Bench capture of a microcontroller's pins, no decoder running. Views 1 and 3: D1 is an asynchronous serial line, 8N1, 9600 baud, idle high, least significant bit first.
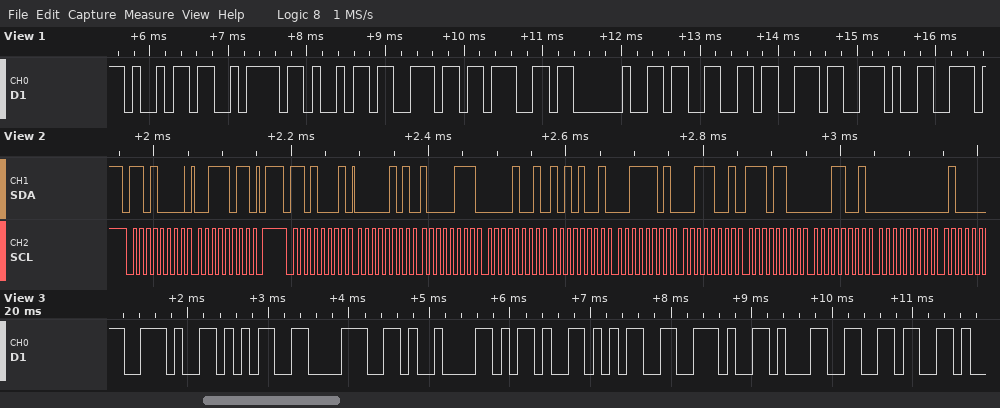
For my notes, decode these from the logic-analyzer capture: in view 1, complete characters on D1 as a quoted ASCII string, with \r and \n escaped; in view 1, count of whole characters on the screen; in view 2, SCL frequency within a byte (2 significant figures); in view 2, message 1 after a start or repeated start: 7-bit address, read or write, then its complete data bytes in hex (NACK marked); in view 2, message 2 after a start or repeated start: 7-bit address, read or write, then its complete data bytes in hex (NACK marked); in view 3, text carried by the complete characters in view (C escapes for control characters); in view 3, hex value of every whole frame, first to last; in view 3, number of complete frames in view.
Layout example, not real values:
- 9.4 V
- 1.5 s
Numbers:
- "izing 3s."
- 9
- 100 kHz
- 0x68 write: 3B
- 0x68 read: 05 87 09 A9 3D 39 EC 19 00
- ".58\t-5.16"
- 2E 35 38 09 2D 35 2E 31 36
- 9
